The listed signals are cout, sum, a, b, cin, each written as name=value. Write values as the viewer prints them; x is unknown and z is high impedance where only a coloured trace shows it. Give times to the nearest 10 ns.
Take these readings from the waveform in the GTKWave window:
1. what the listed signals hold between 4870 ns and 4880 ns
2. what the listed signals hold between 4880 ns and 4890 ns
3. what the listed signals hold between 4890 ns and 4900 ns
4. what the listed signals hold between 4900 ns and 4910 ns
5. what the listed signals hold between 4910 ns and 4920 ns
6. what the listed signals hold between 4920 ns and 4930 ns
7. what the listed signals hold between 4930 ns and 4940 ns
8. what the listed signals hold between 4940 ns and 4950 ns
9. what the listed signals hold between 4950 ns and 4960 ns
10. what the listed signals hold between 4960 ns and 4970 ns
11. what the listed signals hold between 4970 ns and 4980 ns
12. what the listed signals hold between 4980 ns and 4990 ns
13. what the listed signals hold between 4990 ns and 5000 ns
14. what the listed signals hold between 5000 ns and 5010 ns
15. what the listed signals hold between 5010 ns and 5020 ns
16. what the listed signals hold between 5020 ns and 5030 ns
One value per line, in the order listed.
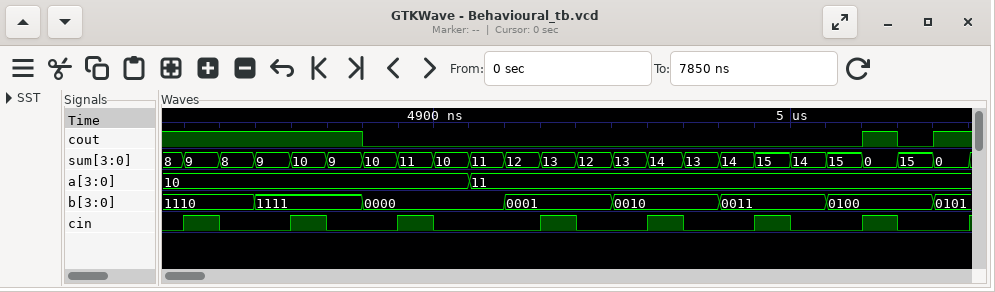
cout=1, sum=9, a=10, b=1111, cin=0
cout=0, sum=10, a=10, b=0000, cin=0
cout=0, sum=11, a=10, b=0000, cin=1
cout=0, sum=10, a=10, b=0000, cin=0
cout=0, sum=11, a=11, b=0000, cin=0
cout=0, sum=12, a=11, b=0001, cin=0
cout=0, sum=13, a=11, b=0001, cin=1
cout=0, sum=12, a=11, b=0001, cin=0
cout=0, sum=13, a=11, b=0010, cin=0
cout=0, sum=14, a=11, b=0010, cin=1
cout=0, sum=13, a=11, b=0010, cin=0
cout=0, sum=14, a=11, b=0011, cin=0
cout=0, sum=15, a=11, b=0011, cin=1
cout=0, sum=14, a=11, b=0011, cin=0
cout=0, sum=15, a=11, b=0100, cin=0
cout=1, sum=0, a=11, b=0100, cin=1
